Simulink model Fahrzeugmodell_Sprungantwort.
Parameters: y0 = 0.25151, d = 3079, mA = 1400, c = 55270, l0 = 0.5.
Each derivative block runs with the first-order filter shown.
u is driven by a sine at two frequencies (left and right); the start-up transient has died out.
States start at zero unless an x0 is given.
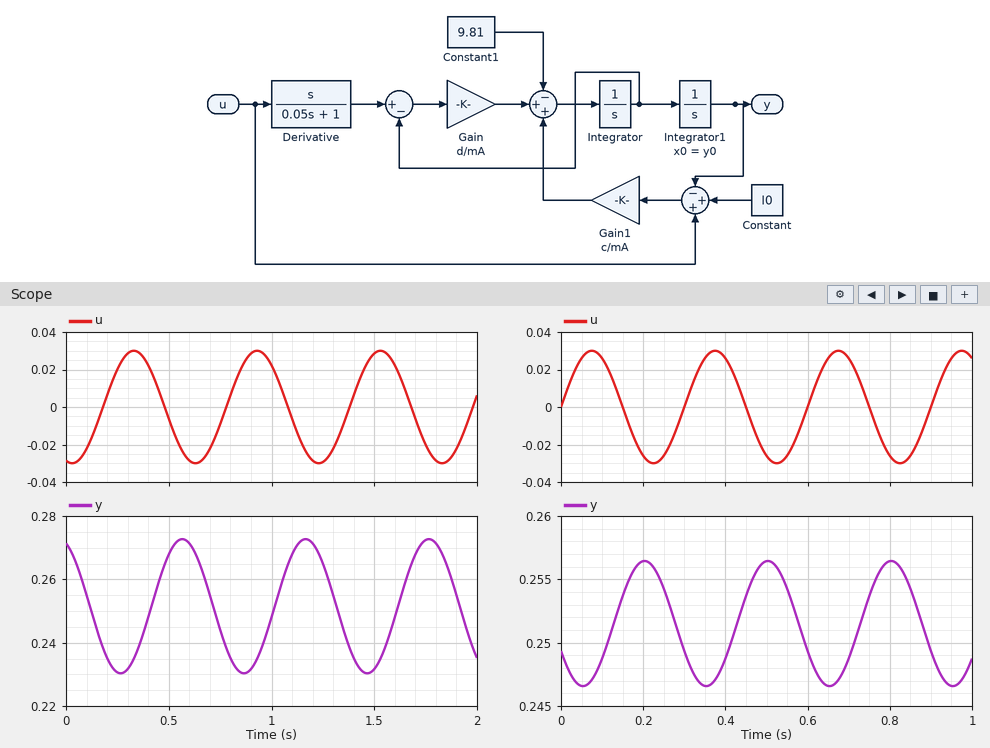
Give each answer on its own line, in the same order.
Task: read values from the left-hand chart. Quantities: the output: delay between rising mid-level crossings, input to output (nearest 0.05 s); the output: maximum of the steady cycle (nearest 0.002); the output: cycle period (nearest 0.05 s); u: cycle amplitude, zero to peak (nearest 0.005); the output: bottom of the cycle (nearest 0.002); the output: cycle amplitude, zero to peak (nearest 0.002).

0.25 s
0.272
0.60 s
0.030
0.230
0.022
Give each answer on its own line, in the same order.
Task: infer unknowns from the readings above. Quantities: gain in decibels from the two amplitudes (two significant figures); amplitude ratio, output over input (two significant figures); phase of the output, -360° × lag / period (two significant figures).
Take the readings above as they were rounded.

-2.7 dB
0.73
-150°
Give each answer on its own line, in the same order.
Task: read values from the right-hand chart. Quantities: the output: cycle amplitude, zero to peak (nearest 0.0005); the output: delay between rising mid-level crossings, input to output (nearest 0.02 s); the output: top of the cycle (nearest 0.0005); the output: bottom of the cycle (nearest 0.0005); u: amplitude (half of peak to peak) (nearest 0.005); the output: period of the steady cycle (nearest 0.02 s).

0.0050
0.12 s
0.2565
0.2465
0.030
0.30 s
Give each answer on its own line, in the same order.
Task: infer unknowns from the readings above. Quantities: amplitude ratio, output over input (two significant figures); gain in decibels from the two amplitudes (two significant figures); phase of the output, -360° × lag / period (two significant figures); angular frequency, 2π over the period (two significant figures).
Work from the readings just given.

0.17
-16 dB
-140°
21 rad/s
